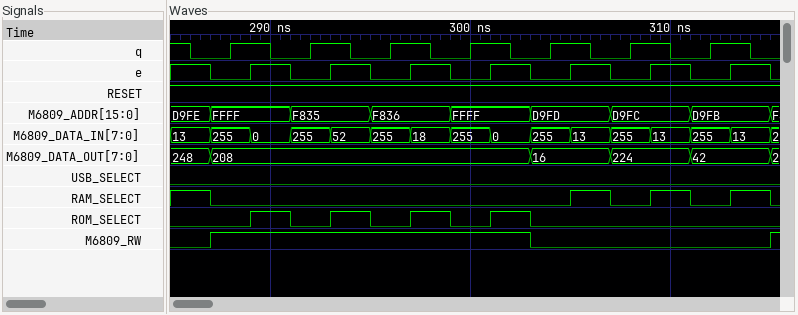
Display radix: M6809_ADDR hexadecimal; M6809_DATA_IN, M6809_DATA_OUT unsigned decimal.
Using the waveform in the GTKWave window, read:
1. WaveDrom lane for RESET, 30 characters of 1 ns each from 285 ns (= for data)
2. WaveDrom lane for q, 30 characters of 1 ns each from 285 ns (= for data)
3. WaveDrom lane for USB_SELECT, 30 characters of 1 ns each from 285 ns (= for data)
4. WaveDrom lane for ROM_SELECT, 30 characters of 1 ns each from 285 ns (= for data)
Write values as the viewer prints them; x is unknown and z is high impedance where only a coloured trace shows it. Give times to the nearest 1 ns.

{name: 'RESET', wave: '1.............................'}
{name: 'q', wave: '10.1.0.1.0.1.0.1.0.1.0.1.0.1.0'}
{name: 'USB_SELECT', wave: '0.............................'}
{name: 'ROM_SELECT', wave: '0...1.0.1.0.1.0.1.0...........'}
